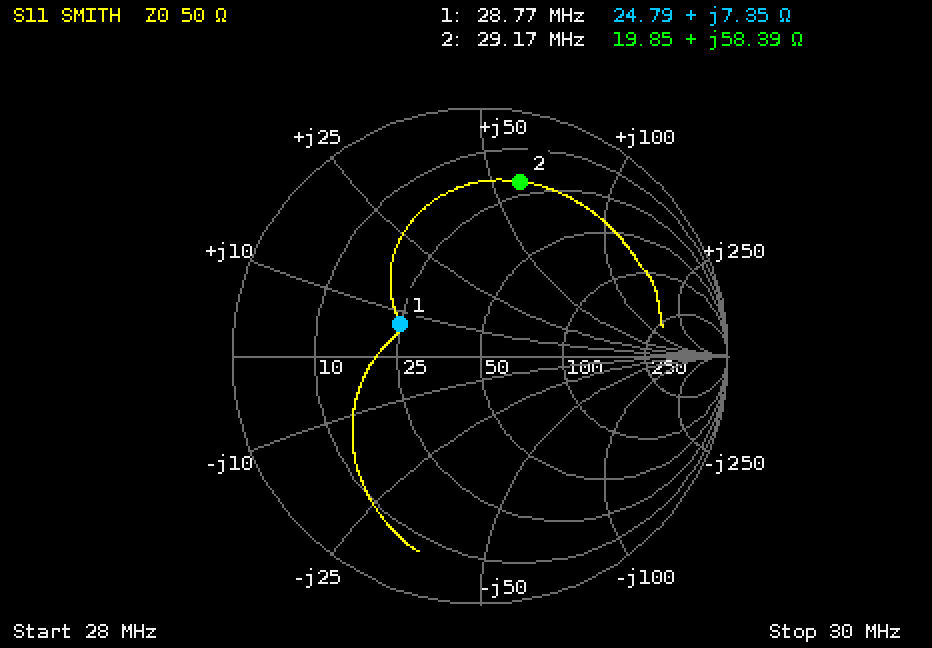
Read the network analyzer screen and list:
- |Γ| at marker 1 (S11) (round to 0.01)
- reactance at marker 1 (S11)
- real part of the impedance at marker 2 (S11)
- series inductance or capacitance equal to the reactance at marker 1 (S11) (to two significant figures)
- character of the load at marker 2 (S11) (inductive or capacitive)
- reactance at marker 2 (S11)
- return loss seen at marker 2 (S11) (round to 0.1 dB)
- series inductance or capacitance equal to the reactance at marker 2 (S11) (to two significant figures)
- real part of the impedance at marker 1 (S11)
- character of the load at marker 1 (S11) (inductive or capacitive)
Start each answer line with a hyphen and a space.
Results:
- 0.35
- +7.35 Ω
- 19.85 Ω
- 41 nH
- inductive
- +58.39 Ω
- 2.8 dB
- 320 nH
- 24.79 Ω
- inductive
